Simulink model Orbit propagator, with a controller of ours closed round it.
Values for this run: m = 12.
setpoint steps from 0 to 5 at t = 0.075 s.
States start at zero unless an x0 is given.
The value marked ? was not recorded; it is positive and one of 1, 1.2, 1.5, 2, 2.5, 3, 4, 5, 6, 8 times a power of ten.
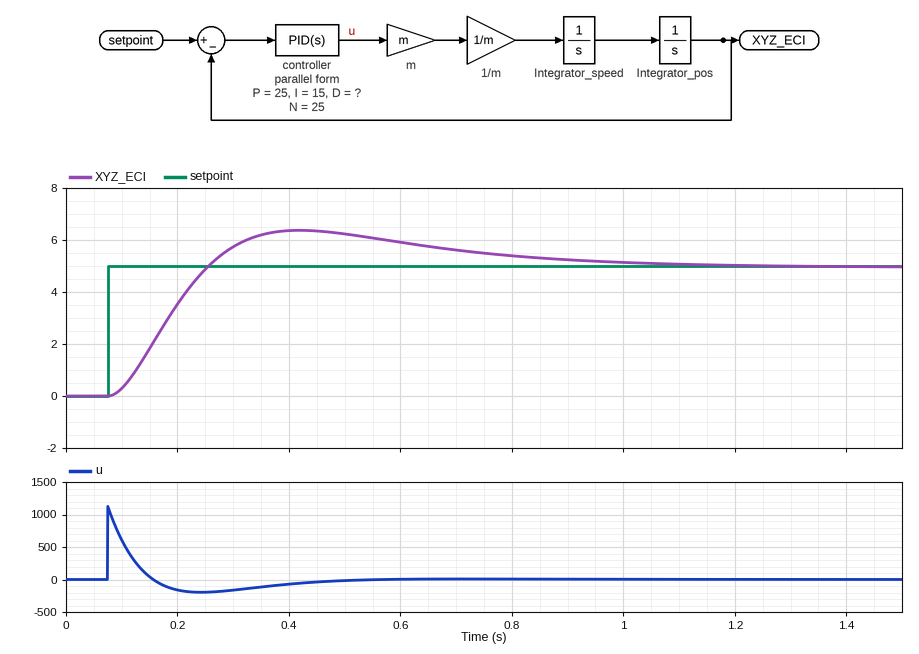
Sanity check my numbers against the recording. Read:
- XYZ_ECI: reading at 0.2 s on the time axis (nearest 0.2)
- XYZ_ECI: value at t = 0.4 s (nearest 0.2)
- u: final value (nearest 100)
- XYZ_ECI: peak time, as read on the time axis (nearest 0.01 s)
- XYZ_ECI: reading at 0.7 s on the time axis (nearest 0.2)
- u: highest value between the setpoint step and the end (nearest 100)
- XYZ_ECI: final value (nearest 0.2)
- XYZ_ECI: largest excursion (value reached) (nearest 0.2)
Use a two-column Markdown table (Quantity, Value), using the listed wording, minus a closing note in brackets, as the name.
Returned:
| Quantity | Value |
|---|---|
| XYZ_ECI: reading at 0.2 s on the time axis | 3.6 |
| XYZ_ECI: value at t = 0.4 s | 6.4 |
| u: final value | 0 |
| XYZ_ECI: peak time, as read on the time axis | 0.42 s |
| XYZ_ECI: reading at 0.7 s on the time axis | 5.6 |
| u: highest value between the setpoint step and the end | 1100 |
| XYZ_ECI: final value | 5.0 |
| XYZ_ECI: largest excursion (value reached) | 6.4 |
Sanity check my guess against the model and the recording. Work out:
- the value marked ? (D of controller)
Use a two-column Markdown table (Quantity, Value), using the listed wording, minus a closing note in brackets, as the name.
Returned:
| Quantity | Value |
|---|---|
| the value marked ? | 8 |
